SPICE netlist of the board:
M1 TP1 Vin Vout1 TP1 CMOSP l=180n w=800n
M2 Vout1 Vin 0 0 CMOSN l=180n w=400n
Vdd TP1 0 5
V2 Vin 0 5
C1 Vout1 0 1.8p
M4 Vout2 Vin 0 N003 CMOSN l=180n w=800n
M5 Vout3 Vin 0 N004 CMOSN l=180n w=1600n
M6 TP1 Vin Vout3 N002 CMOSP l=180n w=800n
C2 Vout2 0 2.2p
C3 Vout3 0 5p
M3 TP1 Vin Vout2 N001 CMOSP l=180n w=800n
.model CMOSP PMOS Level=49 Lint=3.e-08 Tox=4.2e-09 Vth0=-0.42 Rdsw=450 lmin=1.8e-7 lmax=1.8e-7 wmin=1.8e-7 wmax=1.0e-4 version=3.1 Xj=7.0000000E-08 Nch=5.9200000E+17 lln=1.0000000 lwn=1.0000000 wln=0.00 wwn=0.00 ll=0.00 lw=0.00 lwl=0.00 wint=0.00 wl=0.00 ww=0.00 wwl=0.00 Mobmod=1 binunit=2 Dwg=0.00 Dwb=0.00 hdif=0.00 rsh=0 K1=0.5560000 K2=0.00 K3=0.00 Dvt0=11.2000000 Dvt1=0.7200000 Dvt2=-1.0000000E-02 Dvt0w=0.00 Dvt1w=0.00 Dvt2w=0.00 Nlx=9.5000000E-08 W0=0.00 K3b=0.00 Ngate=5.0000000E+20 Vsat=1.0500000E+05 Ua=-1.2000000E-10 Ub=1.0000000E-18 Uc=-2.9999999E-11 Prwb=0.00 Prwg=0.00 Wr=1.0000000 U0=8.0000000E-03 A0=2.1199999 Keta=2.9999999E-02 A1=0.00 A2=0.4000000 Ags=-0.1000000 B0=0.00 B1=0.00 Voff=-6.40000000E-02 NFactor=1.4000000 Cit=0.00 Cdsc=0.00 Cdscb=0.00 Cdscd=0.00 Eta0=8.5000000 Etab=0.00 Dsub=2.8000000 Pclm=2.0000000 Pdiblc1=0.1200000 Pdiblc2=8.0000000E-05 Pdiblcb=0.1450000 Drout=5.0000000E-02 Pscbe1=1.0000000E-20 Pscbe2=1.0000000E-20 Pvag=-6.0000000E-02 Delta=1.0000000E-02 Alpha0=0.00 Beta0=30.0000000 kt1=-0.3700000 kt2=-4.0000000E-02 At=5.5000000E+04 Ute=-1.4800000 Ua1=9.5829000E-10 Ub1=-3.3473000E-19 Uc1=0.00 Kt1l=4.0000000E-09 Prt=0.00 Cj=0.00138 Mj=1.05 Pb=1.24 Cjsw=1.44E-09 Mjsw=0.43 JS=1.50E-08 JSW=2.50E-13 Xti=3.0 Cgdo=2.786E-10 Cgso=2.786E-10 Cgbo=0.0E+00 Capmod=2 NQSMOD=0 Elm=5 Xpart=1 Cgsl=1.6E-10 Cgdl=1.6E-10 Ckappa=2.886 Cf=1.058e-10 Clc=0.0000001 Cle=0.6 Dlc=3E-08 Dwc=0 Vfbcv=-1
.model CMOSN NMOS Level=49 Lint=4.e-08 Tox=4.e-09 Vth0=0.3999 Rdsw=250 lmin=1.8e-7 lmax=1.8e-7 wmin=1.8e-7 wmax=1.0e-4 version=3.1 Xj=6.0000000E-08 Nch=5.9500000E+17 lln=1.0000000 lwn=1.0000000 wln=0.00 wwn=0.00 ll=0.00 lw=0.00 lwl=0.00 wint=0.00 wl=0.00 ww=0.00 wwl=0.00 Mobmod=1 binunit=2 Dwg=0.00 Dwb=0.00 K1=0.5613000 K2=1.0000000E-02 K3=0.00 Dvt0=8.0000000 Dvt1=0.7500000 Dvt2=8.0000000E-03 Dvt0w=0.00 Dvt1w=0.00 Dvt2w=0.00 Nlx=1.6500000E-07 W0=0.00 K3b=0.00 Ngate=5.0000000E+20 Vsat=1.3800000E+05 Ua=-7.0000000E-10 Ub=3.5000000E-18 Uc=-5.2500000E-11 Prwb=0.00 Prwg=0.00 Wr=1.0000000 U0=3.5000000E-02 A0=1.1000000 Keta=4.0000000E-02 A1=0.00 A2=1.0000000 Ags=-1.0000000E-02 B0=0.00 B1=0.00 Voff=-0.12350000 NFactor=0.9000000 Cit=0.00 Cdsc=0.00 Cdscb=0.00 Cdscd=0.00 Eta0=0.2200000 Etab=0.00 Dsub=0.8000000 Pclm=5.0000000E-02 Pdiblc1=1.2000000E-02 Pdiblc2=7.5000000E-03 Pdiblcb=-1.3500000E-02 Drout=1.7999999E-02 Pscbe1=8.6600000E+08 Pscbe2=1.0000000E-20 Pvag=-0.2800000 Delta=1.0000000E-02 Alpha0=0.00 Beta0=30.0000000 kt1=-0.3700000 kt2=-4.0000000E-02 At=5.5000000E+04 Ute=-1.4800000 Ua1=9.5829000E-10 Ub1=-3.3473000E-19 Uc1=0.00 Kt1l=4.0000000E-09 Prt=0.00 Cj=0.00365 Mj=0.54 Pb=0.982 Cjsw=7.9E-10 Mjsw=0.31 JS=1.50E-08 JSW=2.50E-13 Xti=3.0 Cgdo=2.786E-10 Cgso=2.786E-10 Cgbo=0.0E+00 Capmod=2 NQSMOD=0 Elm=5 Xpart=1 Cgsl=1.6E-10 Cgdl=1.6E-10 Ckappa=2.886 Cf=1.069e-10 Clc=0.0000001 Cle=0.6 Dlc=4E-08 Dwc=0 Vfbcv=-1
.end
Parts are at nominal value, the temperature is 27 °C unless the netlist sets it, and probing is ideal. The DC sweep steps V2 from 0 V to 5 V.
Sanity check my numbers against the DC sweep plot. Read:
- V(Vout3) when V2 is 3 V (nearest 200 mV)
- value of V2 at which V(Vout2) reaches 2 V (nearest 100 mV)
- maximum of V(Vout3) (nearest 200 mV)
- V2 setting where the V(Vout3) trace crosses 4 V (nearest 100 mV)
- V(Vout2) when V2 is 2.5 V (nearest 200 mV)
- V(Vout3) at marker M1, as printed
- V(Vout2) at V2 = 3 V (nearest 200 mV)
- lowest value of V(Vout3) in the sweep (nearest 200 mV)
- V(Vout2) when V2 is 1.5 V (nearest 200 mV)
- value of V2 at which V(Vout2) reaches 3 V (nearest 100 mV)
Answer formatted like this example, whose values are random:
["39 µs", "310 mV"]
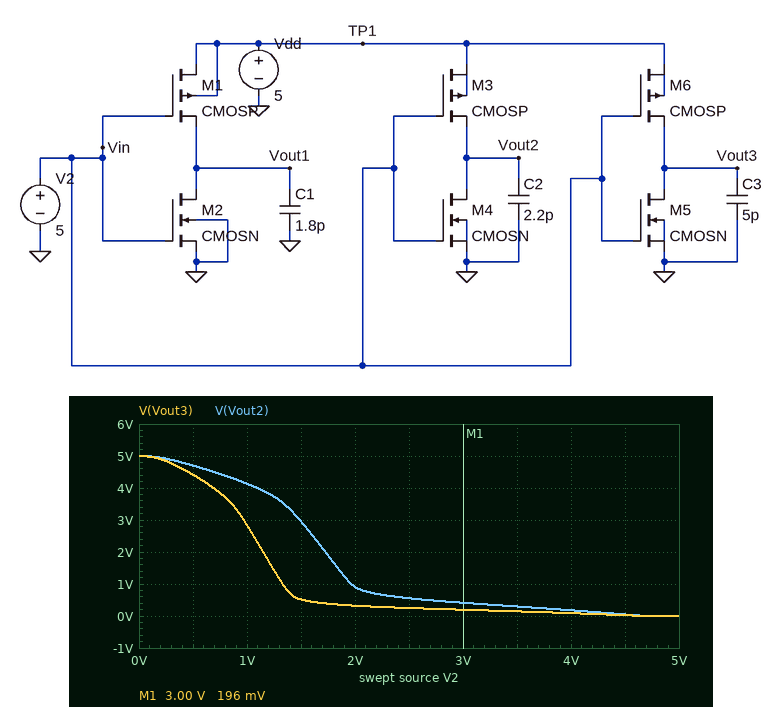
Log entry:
["200 mV", "1.7 V", "5.0 V", "700 mV", "600 mV", "196 mV", "400 mV", "0 V", "3.0 V", "1.5 V"]
